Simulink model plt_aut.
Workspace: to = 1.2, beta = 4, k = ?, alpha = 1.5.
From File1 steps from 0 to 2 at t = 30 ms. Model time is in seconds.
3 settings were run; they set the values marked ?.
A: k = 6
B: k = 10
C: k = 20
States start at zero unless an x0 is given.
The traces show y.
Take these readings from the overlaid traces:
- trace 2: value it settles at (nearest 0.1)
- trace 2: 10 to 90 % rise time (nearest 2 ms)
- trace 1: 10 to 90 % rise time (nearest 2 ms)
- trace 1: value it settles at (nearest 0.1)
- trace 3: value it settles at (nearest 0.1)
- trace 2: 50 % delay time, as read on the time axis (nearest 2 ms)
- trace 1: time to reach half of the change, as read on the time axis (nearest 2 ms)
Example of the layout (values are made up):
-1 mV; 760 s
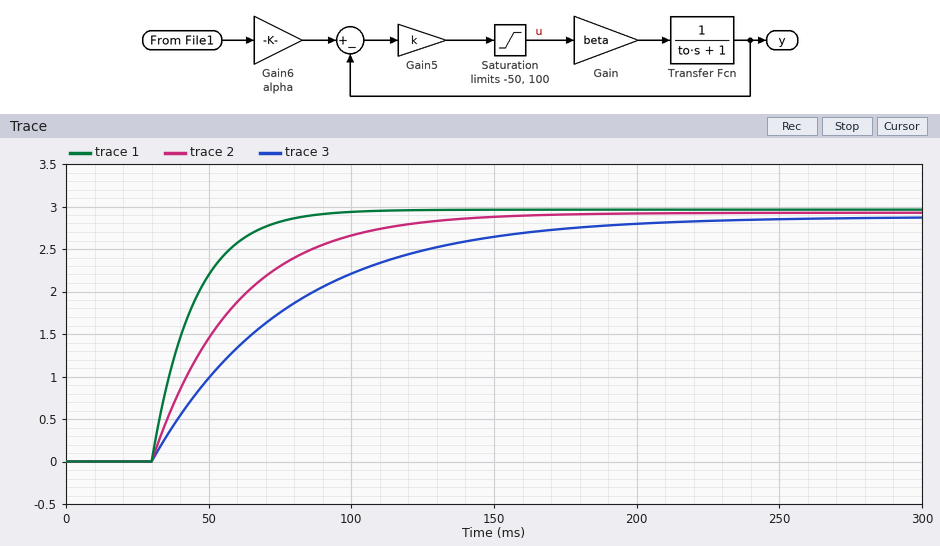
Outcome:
2.9; 64 ms; 32 ms; 3.0; 2.9; 50 ms; 40 ms
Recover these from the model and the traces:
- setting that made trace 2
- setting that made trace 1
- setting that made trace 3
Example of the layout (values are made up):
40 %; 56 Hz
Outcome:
B; C; A
